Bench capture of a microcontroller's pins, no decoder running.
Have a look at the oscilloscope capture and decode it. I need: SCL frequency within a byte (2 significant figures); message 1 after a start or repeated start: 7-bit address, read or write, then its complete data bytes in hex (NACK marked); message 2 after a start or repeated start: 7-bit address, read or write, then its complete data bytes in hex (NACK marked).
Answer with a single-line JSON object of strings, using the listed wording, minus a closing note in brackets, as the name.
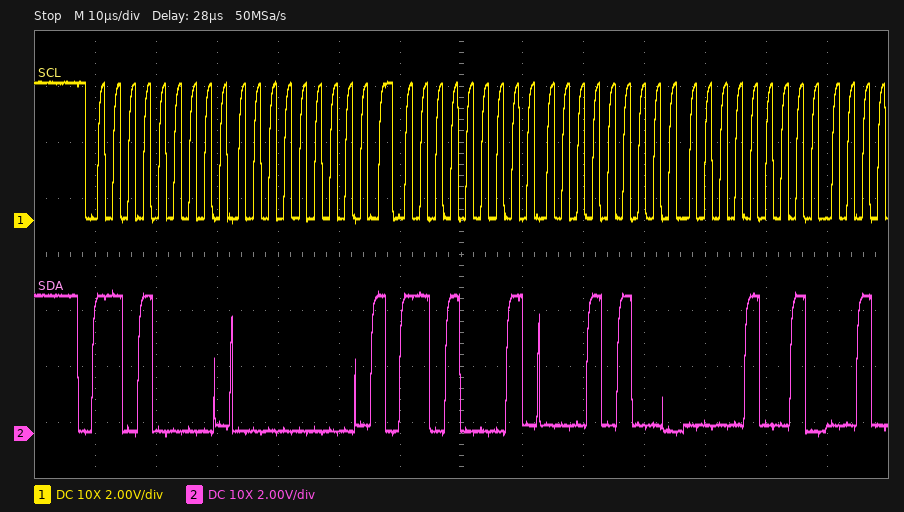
{"SCL frequency within a byte": "400 kHz", "message 1 after a start or repeated start: 7-bit address, read or write, then its complete data bytes in hex": "0x68 write: 00", "message 2 after a start or repeated start: 7-bit address, read or write, then its complete data bytes in hex": "0x68 read: 14 09"}
